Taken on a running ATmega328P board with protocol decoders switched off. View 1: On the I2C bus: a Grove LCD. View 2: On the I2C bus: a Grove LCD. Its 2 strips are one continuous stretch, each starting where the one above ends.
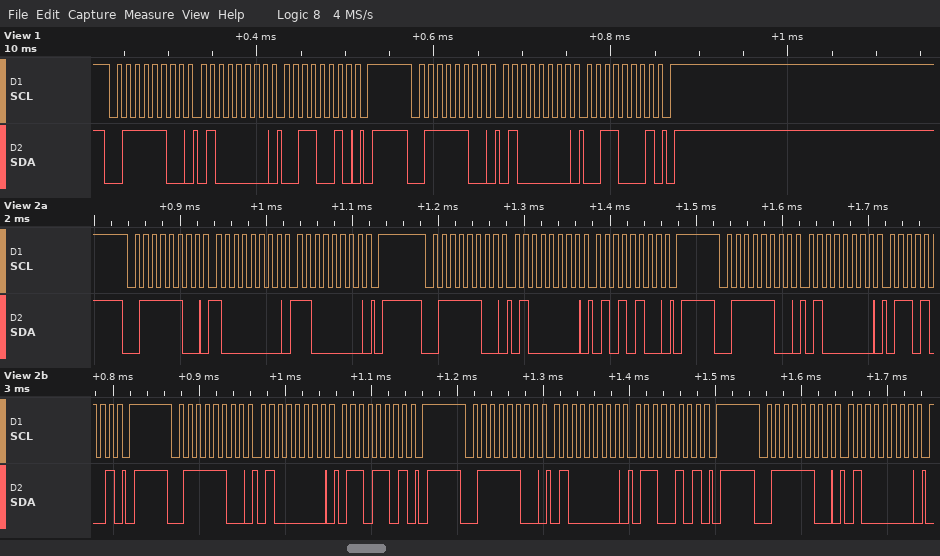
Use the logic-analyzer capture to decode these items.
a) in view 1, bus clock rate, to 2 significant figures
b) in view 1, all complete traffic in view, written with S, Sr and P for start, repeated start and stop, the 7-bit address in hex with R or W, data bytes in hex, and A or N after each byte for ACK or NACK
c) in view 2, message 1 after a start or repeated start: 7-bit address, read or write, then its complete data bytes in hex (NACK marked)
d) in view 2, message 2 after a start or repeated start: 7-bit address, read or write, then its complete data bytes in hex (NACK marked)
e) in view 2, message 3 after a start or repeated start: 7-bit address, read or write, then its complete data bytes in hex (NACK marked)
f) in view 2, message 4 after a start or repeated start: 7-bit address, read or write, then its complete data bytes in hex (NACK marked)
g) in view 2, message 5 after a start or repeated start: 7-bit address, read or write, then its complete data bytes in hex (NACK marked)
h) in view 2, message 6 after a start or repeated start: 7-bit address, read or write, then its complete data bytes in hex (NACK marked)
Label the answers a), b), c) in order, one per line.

a) 100 kHz
b) S 3EW A 40 A 32 A P S 3EW A 40 A 31 A P
c) 0x3E write: 80 C0
d) 0x3E write: 40 54
e) 0x3E write: 40 69
f) 0x3E write: 40 6D
g) 0x3E write: 40 65
h) 0x3E write: 40
